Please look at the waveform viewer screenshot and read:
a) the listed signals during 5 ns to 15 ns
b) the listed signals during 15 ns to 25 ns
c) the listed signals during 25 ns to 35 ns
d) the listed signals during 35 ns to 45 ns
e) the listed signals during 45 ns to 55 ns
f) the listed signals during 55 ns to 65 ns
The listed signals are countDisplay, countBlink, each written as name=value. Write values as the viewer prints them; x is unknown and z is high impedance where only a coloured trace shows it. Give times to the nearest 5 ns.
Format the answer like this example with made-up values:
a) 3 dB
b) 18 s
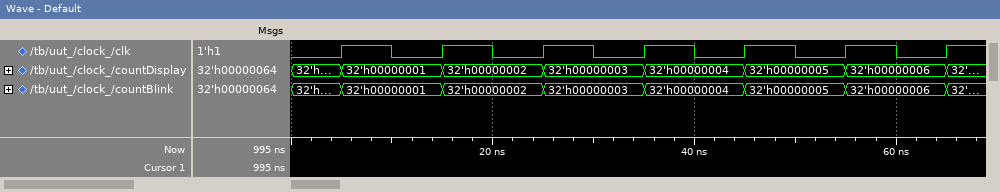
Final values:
a) countDisplay=32'h00000001, countBlink=32'h00000001
b) countDisplay=32'h00000002, countBlink=32'h00000002
c) countDisplay=32'h00000003, countBlink=32'h00000003
d) countDisplay=32'h00000004, countBlink=32'h00000004
e) countDisplay=32'h00000005, countBlink=32'h00000005
f) countDisplay=32'h00000006, countBlink=32'h00000006
